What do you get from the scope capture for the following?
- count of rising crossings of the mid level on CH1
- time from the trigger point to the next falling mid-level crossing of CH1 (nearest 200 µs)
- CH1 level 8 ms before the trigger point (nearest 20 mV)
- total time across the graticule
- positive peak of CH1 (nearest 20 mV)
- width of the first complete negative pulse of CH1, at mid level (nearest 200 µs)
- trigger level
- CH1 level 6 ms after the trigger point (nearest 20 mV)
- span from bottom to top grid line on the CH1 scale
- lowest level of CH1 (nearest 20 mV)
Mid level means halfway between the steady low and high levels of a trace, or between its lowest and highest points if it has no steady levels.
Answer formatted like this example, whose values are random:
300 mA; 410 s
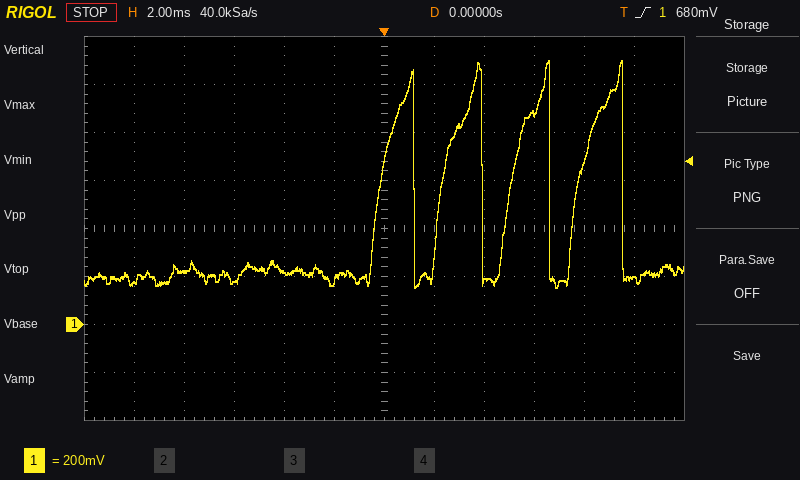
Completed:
4; 1.2 ms; 220 mV; 24 ms; 1.10 V; 1.2 ms; 680 mV; 880 mV; 1.6 V; 160 mV
